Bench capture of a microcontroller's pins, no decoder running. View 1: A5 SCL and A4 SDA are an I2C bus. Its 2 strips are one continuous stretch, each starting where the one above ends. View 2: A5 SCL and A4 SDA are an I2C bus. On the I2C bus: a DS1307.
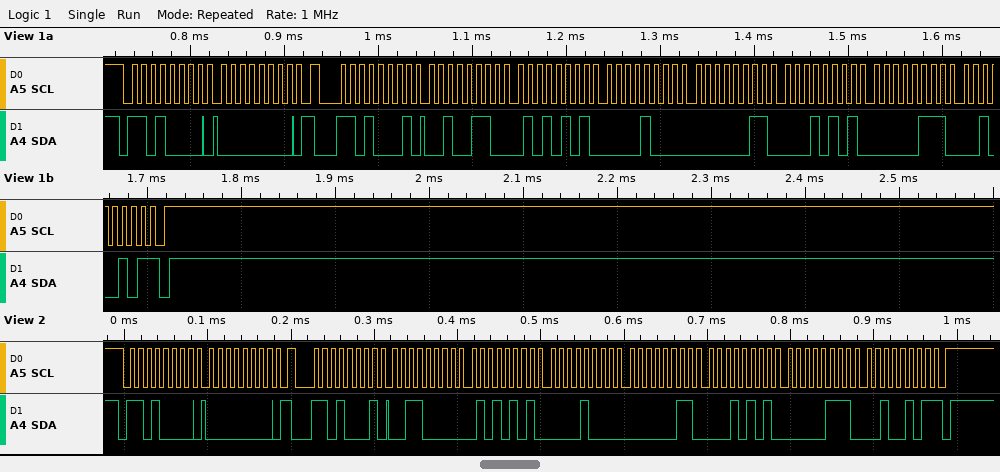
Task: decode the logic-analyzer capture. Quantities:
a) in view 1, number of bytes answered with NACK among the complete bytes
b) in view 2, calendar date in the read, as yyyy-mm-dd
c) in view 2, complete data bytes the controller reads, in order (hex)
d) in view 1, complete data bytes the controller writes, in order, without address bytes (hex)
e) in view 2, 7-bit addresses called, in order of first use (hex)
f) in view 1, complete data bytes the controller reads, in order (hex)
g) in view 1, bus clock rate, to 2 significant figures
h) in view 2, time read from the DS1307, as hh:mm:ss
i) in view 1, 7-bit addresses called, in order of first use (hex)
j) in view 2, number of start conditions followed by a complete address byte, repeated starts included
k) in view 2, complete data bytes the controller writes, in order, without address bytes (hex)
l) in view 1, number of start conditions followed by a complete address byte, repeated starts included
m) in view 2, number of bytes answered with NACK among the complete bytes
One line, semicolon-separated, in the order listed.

1; 2025-07-15; 30 55 08 03 15 07 25; 00; 0x68; 26 55 08 03 15 07 25; 100 kHz; 08:55:30; 0x68; 2; 00; 2; 1
